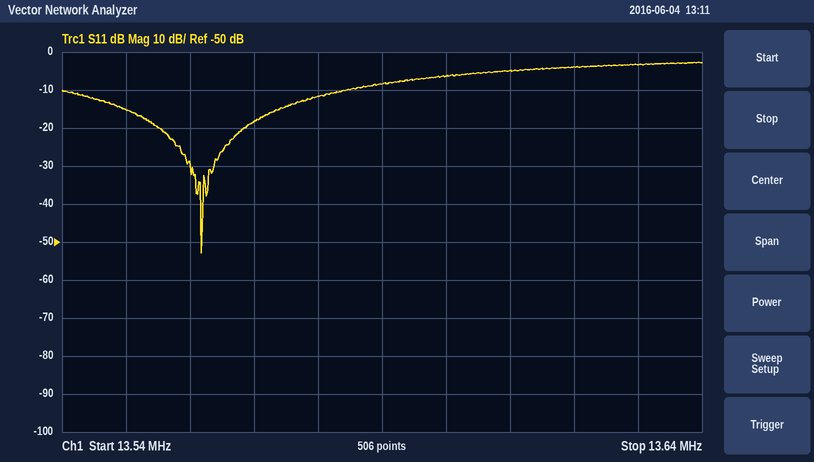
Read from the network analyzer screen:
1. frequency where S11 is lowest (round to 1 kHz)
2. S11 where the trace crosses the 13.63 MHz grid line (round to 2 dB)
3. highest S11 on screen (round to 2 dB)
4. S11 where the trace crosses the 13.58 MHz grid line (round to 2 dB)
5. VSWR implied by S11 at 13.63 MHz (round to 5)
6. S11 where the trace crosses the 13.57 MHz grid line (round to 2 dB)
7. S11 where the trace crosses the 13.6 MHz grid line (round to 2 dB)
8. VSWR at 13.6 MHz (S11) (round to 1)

13.562 MHz
-4 dB
-2 dB
-12 dB
5
-18 dB
-6 dB
3
